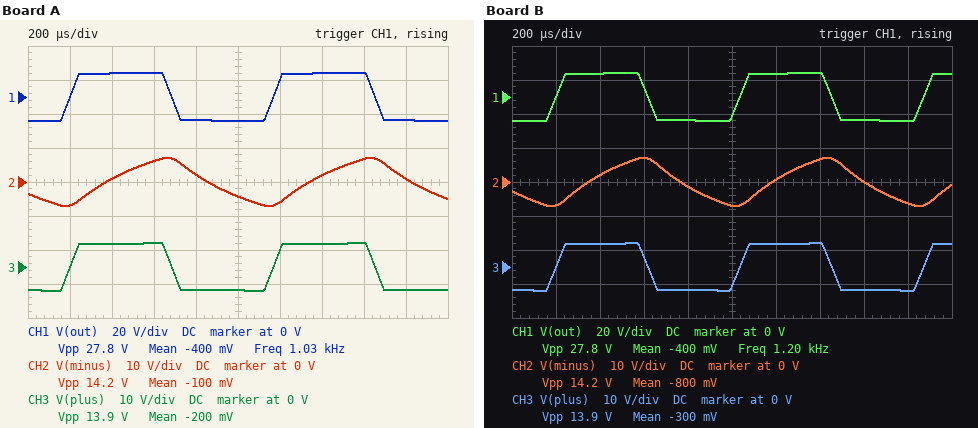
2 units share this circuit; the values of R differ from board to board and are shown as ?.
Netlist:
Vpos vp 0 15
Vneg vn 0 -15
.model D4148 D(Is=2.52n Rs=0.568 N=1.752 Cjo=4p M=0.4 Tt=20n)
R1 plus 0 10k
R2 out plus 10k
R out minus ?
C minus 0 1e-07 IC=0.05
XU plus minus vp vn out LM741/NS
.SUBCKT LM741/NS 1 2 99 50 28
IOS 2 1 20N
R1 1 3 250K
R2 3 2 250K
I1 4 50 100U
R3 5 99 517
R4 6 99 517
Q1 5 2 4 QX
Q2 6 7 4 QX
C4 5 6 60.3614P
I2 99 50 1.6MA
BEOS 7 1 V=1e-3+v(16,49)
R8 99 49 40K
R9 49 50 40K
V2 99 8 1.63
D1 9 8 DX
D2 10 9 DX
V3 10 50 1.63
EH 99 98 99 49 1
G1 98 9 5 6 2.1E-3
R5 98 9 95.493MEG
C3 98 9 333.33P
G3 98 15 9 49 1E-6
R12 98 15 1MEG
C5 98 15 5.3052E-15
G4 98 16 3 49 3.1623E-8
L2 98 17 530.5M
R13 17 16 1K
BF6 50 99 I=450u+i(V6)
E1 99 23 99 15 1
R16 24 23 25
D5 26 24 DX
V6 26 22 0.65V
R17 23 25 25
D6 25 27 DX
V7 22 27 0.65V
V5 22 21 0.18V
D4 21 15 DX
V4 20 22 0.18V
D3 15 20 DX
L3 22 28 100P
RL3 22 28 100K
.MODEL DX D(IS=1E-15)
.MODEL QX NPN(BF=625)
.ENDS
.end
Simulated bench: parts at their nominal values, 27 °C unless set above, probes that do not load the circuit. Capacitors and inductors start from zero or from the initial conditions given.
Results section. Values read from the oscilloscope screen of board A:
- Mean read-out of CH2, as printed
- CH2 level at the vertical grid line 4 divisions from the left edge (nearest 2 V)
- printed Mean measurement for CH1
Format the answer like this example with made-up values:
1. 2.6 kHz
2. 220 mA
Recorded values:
1. -100 mV
2. 2 V
3. -400 mV
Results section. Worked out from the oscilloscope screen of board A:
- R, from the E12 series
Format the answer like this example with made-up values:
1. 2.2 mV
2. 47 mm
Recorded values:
1. 3.9 kΩ
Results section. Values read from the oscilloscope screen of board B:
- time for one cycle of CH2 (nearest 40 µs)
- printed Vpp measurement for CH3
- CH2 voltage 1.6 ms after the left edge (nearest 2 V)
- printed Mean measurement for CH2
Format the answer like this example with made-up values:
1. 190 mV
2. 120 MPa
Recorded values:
1. 840 µs
2. 13.9 V
3. 0 V
4. -800 mV
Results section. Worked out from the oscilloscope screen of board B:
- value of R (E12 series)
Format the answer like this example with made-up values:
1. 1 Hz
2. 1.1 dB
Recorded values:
1. 3.3 kΩ
